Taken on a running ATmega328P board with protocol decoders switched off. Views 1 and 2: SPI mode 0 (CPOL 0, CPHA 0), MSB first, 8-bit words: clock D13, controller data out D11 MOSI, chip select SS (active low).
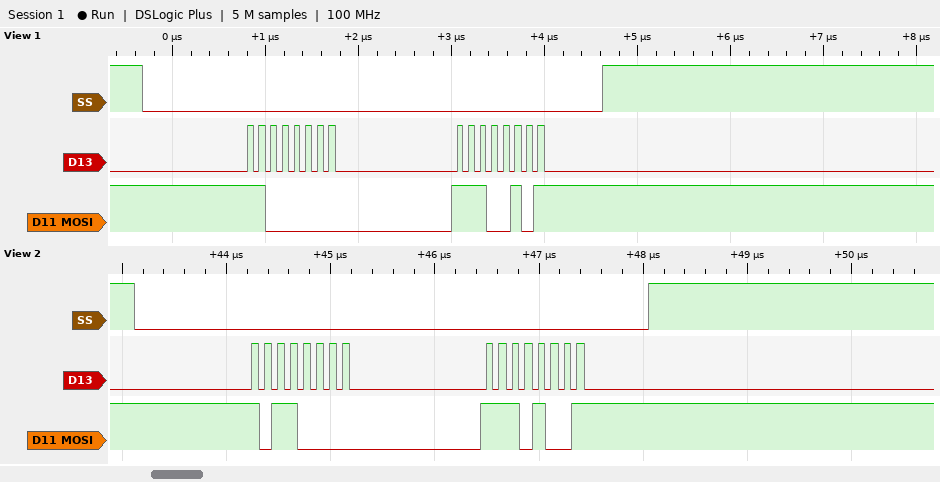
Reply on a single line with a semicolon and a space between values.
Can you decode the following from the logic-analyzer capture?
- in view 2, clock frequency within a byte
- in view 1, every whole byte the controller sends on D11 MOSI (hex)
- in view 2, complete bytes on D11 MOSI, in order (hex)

8 MHz; C0 E5; 0xB0 0xE9
